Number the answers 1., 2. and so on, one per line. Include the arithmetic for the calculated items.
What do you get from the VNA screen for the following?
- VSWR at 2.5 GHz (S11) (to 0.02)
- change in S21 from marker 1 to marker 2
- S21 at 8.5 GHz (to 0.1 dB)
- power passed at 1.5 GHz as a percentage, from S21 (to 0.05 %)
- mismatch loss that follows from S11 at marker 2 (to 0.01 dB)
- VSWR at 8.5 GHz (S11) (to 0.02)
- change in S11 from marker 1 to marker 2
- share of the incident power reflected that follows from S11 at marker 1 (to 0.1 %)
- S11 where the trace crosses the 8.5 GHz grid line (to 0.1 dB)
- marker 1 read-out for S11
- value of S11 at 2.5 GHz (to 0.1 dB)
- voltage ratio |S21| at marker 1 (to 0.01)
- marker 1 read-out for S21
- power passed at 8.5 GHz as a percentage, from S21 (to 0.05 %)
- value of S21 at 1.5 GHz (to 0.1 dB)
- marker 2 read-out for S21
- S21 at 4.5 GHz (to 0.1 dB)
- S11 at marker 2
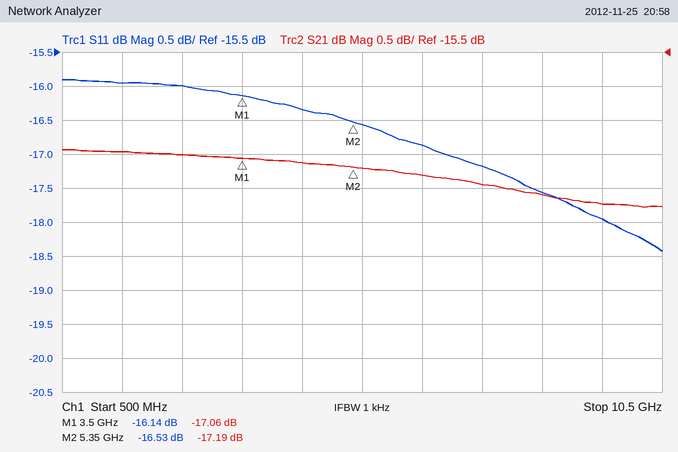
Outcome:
1. |Γ| = 10^(-16/20) = 0.1585; VSWR = (1 + 0.1585)/(1 − 0.1585) ≈ 1.38
2. -17.19 − (-17.06) = -0.13 dB
3. -17.6 dB
4. 10^(-17/10) ≈ 2.00 %
5. −10 log10(1 − 10^(-16.53/10)) ≈ 0.10 dB
6. |Γ| = 10^(-17.6/20) = 0.1318; VSWR = (1 + 0.1318)/(1 − 0.1318) ≈ 1.30
7. -16.53 − (-16.14) = -0.39 dB
8. 10^(-16.14/10) ≈ 2.4 %
9. -17.6 dB
10. -16.14 dB
11. -16.0 dB
12. 10^(-17.06/20) ≈ 0.14
13. -17.06 dB
14. 10^(-17.6/10) ≈ 1.74 %, so 1.75 % to the nearest 0.05 %
15. -17.0 dB
16. -17.19 dB
17. -17.1 dB
18. -16.53 dB
